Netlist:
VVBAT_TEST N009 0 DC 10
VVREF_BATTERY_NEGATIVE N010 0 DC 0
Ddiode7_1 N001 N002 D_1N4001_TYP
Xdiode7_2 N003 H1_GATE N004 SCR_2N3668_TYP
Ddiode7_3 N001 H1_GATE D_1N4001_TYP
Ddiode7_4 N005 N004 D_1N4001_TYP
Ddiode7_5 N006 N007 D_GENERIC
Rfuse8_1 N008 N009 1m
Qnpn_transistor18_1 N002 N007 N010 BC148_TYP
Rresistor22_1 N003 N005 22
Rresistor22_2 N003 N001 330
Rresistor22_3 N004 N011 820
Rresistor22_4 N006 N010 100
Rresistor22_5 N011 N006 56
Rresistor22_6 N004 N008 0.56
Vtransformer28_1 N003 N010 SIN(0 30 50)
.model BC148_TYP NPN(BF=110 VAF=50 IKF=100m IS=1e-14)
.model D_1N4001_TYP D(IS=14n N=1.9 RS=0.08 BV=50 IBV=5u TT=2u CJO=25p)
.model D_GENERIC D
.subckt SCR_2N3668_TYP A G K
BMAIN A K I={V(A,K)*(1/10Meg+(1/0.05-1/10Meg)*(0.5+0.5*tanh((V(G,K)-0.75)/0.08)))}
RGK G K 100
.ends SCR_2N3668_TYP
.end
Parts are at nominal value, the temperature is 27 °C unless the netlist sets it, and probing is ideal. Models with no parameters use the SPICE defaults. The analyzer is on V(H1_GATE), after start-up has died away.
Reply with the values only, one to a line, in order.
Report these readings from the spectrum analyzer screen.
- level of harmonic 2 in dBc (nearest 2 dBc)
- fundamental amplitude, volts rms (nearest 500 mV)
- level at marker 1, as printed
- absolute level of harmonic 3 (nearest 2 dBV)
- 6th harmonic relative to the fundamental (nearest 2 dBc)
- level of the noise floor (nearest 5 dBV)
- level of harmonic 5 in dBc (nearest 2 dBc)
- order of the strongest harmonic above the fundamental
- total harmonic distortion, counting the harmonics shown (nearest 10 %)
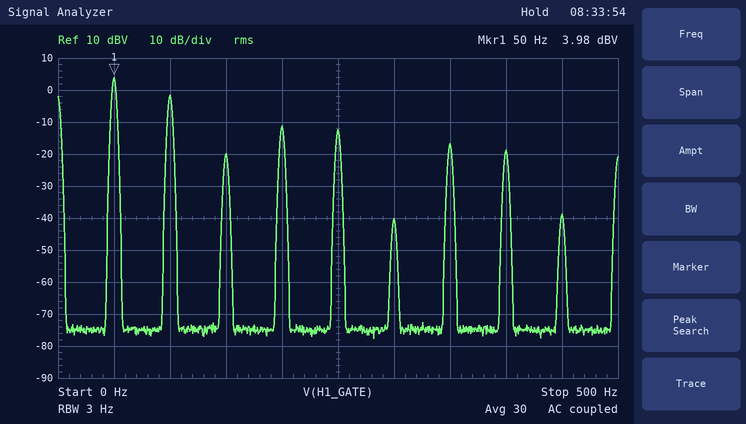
-6 dBc
1.5 V
3.98 dBV
-20 dBV
-44 dBc
-75 dBV
-16 dBc
2
60 %
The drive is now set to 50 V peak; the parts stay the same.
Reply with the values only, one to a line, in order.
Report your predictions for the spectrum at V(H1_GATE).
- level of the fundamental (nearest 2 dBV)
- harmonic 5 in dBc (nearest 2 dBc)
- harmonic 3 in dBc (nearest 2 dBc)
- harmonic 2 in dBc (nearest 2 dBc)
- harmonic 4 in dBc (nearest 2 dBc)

8 dBV
-30 dBc
-26 dBc
-14 dBc
-12 dBc
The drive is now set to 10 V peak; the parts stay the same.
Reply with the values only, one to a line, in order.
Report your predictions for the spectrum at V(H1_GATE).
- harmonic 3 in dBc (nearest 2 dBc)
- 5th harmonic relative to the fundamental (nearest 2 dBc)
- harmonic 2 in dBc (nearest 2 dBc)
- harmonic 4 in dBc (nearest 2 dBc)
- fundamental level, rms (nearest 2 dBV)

-18 dBc
-28 dBc
-12 dBc
-24 dBc
-114 dBV
